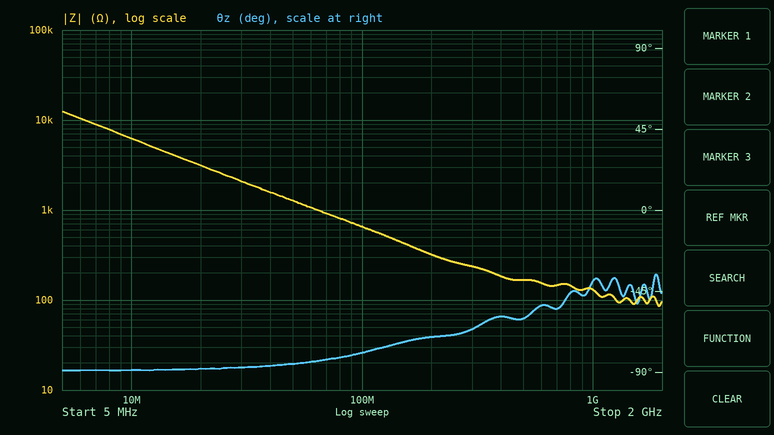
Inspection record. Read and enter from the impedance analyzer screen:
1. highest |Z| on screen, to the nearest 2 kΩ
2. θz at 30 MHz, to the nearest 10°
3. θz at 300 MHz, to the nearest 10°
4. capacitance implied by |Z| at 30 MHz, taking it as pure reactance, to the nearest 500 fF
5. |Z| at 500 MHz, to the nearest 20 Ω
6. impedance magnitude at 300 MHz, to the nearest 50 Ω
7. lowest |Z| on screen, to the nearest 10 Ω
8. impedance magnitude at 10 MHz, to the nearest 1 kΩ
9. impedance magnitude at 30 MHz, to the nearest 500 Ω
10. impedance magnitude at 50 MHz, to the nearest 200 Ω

12 kΩ
-90°
-70°
2.5 pF
160 Ω
250 Ω
90 Ω
6 kΩ
2.0 kΩ
1.2 kΩ
